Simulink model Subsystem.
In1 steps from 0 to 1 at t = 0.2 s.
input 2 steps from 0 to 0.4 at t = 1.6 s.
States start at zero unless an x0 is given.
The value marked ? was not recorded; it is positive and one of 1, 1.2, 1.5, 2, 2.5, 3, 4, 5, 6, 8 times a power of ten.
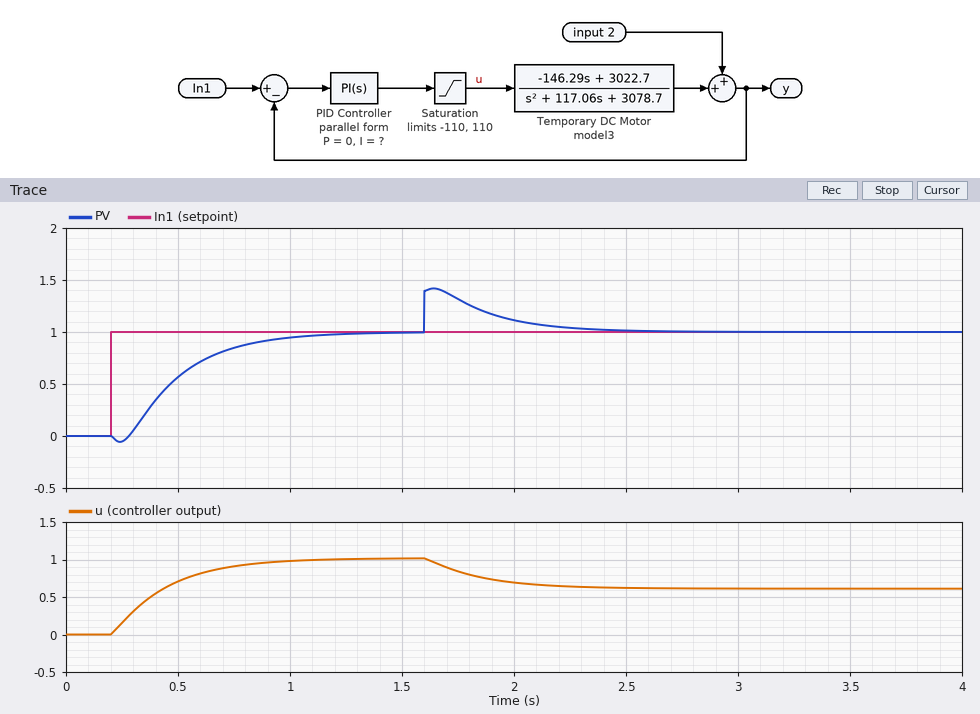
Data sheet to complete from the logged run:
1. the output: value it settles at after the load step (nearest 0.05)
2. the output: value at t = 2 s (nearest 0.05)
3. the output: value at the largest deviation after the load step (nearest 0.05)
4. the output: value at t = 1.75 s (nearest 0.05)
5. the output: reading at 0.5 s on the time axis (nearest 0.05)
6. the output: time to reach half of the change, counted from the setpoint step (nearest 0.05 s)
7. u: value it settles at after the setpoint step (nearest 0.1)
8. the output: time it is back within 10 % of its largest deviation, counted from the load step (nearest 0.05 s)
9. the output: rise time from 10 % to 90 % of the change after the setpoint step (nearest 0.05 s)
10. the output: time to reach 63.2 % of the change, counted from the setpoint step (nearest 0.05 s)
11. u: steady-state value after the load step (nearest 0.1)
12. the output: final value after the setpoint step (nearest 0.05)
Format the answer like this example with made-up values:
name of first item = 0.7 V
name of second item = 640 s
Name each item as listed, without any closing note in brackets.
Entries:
the output: value it settles at after the load step = 1.00
the output: value at t = 2 s = 1.10
the output: value at the largest deviation after the load step = 1.40
the output: value at t = 1.75 s = 1.30
the output: reading at 0.5 s on the time axis = 0.55
the output: time to reach half of the change, counted from the setpoint step = 0.25 s
u: value it settles at after the setpoint step = 1.0
the output: time it is back within 10 % of its largest deviation, counted from the load step = 0.65 s
the output: rise time from 10 % to 90 % of the change after the setpoint step = 0.55 s
the output: time to reach 63.2 % of the change, counted from the setpoint step = 0.35 s
u: steady-state value after the load step = 0.6
the output: final value after the setpoint step = 1.00
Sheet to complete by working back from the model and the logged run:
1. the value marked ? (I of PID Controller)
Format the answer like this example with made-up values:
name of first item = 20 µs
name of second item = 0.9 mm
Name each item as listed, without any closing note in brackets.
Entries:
the value marked ? = 3
